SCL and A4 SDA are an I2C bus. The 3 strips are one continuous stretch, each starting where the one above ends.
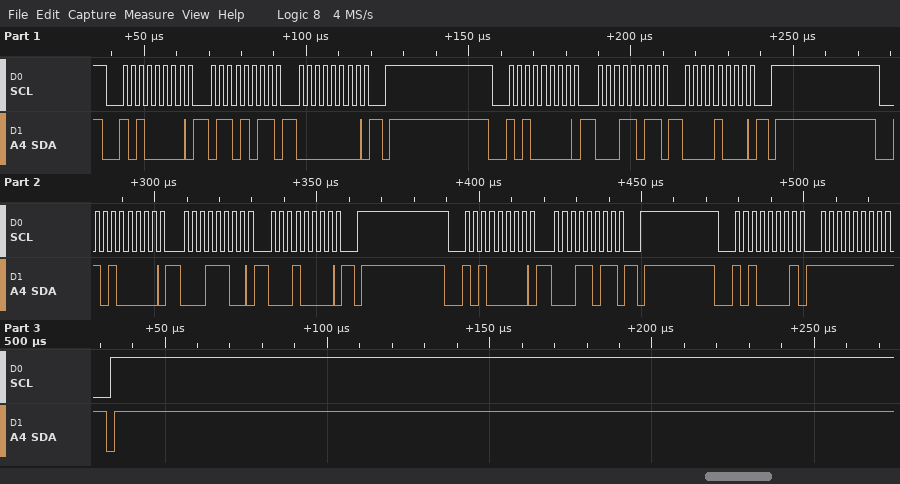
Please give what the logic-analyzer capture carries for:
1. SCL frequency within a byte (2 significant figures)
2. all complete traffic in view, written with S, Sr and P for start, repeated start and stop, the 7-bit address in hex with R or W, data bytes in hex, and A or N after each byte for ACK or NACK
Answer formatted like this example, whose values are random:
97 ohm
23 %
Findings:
400 kHz
S 50W A 6B A 00 A P S 50W A 1B A 08 A P S 50W A 1C A 10 A P S 50W A 1B A P S 50R A FF N P
